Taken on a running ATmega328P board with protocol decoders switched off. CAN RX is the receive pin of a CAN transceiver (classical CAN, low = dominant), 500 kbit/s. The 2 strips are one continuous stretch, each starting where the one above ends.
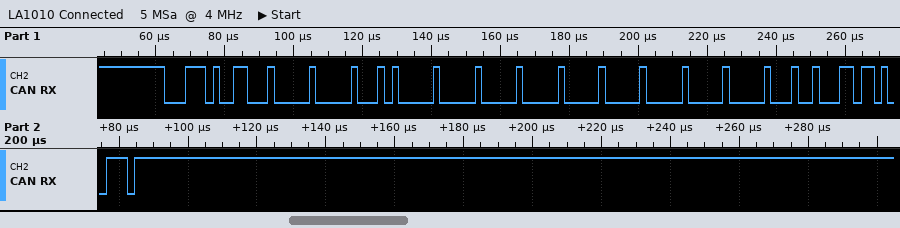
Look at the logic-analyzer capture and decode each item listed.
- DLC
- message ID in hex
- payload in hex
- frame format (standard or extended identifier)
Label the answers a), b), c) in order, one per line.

a) 8
b) 0x1D3
c) 00 28 00 00 00 00 00 04
d) standard
